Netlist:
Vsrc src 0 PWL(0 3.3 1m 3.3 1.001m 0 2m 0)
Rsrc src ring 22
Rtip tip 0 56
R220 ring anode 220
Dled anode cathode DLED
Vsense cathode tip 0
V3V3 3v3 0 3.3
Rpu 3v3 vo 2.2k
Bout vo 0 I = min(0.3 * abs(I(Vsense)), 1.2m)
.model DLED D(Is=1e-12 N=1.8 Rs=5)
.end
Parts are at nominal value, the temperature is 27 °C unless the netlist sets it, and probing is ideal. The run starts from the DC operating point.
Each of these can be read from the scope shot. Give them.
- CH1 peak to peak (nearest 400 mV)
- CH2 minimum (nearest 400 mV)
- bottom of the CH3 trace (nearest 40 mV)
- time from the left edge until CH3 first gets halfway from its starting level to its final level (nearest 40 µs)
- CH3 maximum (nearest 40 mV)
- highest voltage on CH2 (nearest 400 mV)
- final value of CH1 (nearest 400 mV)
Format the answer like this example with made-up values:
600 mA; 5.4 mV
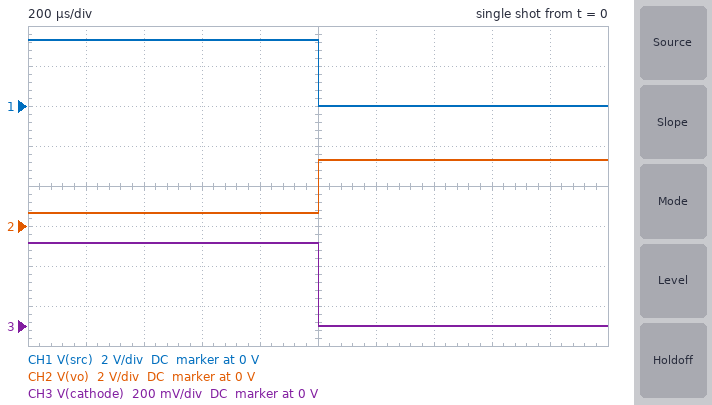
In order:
3.2 V; 800 mV; 0 V; 1.00 ms; 400 mV; 3.2 V; 0 V
